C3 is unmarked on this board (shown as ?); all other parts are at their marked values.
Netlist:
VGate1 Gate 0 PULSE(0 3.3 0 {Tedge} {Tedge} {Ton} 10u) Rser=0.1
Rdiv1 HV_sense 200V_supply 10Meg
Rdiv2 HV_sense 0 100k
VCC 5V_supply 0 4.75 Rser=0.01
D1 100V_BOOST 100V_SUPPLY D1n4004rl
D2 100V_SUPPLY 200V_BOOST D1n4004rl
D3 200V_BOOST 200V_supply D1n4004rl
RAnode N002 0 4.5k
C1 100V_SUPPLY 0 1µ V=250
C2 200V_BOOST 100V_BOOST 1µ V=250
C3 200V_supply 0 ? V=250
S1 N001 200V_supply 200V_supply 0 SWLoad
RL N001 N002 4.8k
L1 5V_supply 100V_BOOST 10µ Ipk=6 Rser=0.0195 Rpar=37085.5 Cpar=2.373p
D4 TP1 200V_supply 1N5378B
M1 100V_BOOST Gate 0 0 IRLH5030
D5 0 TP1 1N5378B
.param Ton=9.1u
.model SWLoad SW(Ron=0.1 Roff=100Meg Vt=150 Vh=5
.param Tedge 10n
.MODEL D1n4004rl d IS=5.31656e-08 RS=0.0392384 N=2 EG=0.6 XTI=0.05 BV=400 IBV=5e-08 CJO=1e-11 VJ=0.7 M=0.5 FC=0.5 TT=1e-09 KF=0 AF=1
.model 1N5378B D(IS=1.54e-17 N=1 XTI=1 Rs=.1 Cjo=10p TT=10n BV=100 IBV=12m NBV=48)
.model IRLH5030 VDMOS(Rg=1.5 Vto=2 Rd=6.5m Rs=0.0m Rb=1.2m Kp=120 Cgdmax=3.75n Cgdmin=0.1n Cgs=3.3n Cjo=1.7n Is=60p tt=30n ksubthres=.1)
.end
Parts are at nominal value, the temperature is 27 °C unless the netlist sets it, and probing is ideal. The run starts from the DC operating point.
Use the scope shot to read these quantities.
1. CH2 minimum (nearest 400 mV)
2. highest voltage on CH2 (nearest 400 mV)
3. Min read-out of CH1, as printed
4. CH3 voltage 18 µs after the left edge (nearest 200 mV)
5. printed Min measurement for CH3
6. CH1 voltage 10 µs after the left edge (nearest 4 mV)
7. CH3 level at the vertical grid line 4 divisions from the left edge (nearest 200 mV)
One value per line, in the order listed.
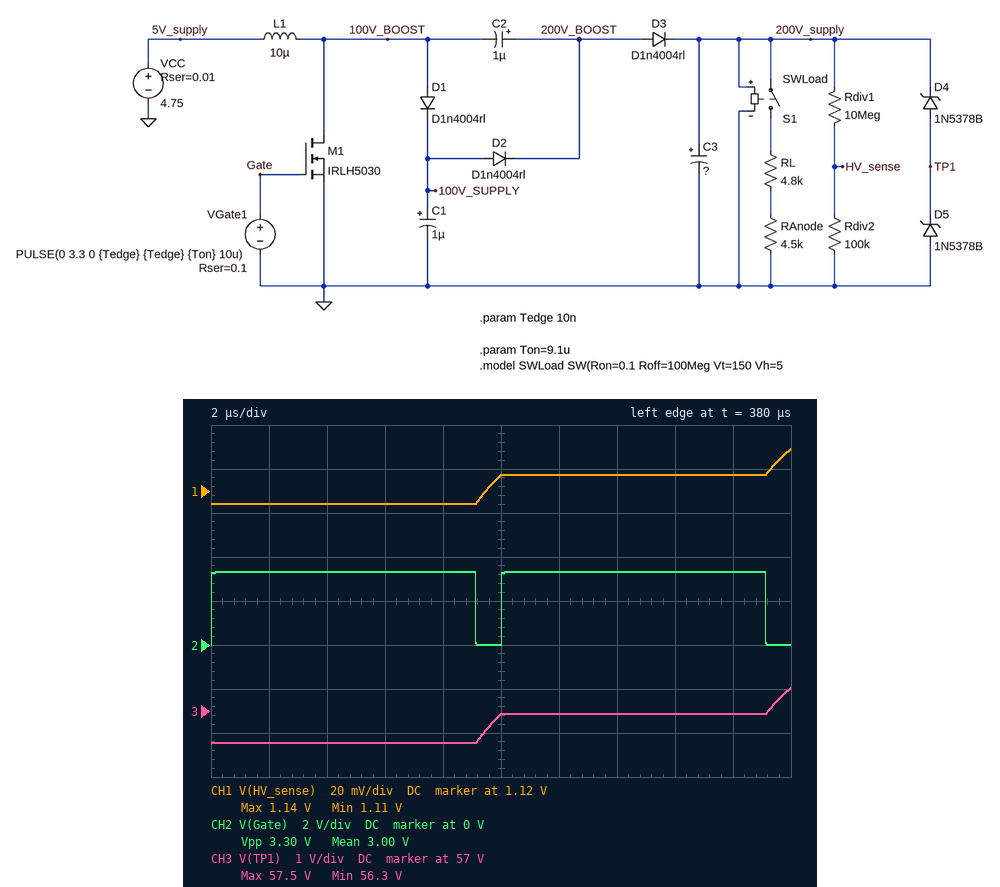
0 V
3.2 V
1.11 V
57.0 V
56.3 V
1.128 V
56.2 V
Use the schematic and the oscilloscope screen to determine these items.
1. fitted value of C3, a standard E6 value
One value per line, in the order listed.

3.3 µF
